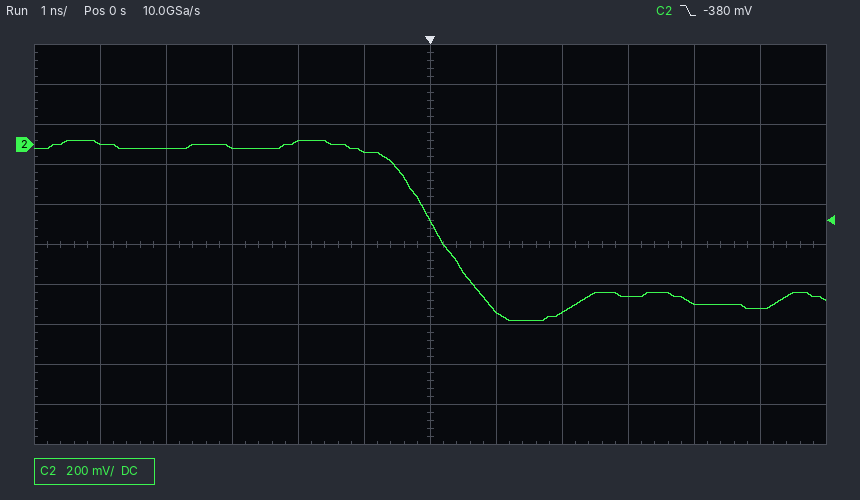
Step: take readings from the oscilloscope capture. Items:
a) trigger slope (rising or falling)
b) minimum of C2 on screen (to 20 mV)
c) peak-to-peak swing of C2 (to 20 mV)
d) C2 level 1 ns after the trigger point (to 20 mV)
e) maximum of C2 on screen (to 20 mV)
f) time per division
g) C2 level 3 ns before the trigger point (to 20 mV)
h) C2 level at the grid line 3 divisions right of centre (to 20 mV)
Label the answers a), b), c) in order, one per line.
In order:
a) falling
b) -880 mV
c) 900 mV
d) -840 mV
e) 20 mV
f) 1 ns
g) -20 mV
h) -760 mV
